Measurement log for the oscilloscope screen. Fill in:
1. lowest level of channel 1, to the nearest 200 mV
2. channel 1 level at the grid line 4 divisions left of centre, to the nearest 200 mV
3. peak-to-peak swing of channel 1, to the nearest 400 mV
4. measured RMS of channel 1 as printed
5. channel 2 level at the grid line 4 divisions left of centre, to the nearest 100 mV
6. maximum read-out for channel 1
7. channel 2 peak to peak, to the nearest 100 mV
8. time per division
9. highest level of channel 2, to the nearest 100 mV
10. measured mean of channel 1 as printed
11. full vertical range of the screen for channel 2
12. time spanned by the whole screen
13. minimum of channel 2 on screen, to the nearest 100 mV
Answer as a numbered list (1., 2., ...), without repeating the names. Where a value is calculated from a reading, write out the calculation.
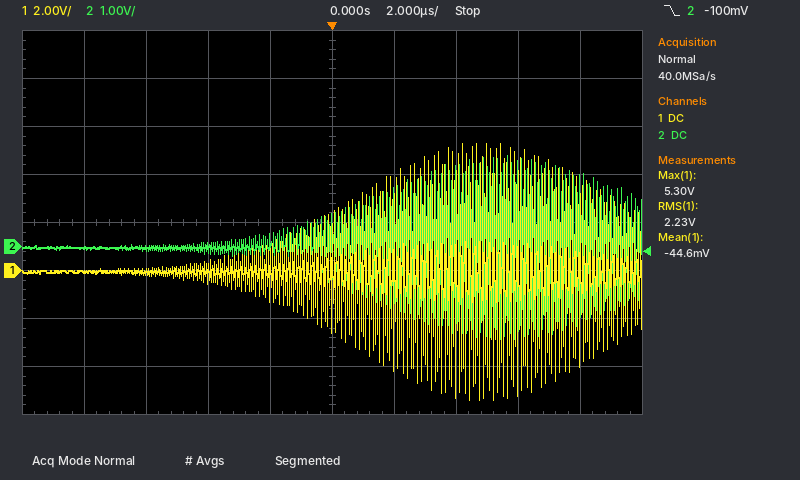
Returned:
1. -5.4 V
2. 0.0 V
3. 10.8 V
4. 2.23 V
5. 0.0 V
6. 5.30 V
7. 1.9 V − (-1.9 V) = 3.8 V
8. 2 µs
9. 1.9 V
10. -44.6 mV
11. 8 V
12. 20 µs
13. -1.9 V
